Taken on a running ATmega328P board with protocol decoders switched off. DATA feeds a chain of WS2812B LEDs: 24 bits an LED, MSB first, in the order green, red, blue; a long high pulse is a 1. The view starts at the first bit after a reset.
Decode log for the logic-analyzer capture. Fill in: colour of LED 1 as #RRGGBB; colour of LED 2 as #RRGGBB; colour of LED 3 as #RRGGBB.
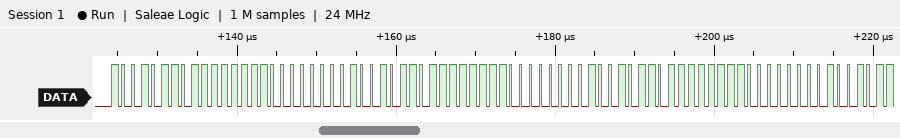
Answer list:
#FF9600
#FF9600
#FF9600
